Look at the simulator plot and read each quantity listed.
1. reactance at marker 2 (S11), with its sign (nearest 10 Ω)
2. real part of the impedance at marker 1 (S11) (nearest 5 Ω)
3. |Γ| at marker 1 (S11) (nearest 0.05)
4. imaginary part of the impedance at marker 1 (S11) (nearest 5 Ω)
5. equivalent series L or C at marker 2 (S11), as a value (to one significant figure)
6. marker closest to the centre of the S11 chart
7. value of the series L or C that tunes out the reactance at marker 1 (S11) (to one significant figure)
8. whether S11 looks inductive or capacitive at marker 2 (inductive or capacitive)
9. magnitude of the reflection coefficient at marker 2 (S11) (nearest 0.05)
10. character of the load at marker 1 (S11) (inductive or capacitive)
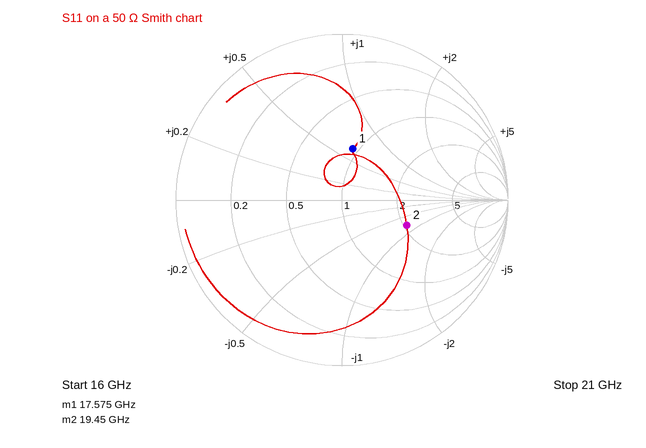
-40 Ω
45 Ω
0.30
+30 Ω
200 fF
marker 1
300 fF
capacitive
0.40
inductive
